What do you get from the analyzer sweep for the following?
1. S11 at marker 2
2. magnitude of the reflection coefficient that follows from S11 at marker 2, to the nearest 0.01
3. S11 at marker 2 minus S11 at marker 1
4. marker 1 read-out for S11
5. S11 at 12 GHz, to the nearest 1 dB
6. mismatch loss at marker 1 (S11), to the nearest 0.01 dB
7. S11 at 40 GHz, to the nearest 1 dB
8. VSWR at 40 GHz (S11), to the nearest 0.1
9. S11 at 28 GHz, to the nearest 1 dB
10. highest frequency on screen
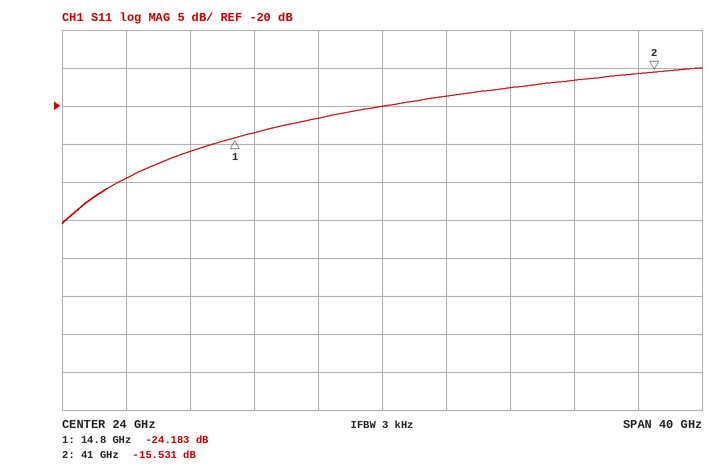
-15.531 dB
0.17
8.652 dB
-24.183 dB
-26 dB
0.02 dB
-16 dB
1.4
-19 dB
44 GHz
